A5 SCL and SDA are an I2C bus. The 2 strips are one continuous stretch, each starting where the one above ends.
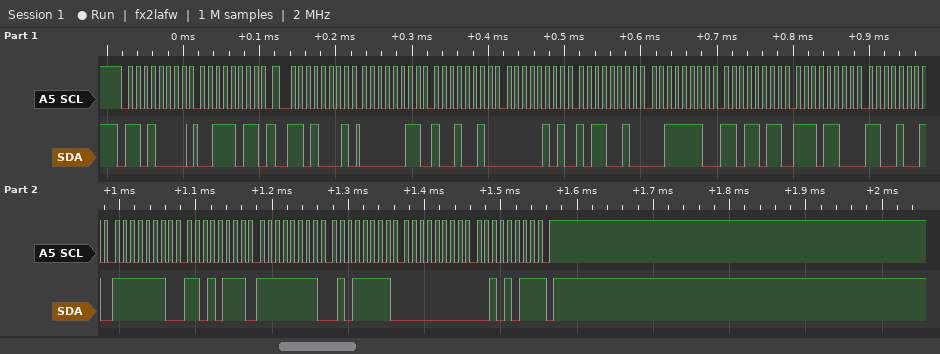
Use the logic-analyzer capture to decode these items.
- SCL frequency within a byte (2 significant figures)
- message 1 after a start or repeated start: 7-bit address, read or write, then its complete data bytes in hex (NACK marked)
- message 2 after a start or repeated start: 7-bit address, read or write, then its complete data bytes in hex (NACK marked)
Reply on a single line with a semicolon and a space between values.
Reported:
100 kHz; 0x68 write: 3B; 0x68 read: 03 92 05 B2 3E DB EC C9 FE D7 FF 5F 00 2B NACK
